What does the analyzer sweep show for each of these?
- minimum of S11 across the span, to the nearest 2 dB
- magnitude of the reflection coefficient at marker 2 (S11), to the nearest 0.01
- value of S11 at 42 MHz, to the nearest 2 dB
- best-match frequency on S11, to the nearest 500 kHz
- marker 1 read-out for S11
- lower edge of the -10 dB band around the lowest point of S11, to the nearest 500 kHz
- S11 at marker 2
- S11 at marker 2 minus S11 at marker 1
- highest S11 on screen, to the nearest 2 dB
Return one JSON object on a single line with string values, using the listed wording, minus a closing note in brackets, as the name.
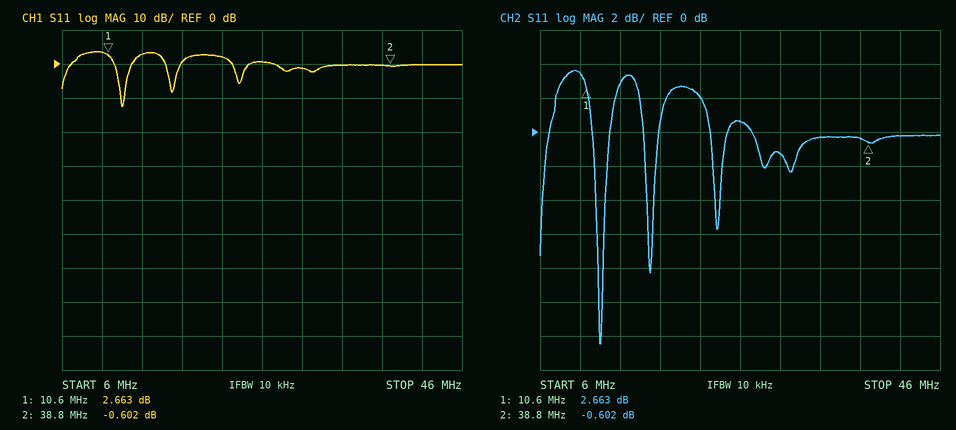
{"minimum of S11 across the span, to the nearest 2 dB": "-12 dB", "magnitude of the reflection coefficient at marker 2 (S11), to the nearest 0.01": "0.93", "value of S11 at 42 MHz, to the nearest 2 dB": "0 dB", "best-match frequency on S11, to the nearest 500 kHz": "12.0 MHz", "marker 1 read-out for S11": "2.663 dB", "lower edge of the -10 dB band around the lowest point of S11, to the nearest 500 kHz": "12.0 MHz", "S11 at marker 2": "-0.602 dB", "S11 at marker 2 minus S11 at marker 1": "-3.265 dB", "highest S11 on screen, to the nearest 2 dB": "4 dB"}
